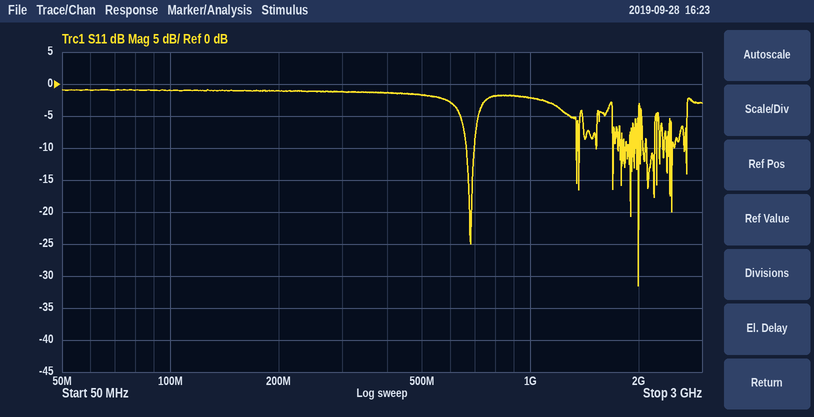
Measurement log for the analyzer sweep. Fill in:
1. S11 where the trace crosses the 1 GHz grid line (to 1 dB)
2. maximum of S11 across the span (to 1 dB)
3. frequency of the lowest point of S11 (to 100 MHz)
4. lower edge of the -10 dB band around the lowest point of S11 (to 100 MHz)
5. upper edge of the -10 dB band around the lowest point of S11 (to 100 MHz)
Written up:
-2 dB
-1 dB
2.0 GHz
2.0 GHz
2.0 GHz
